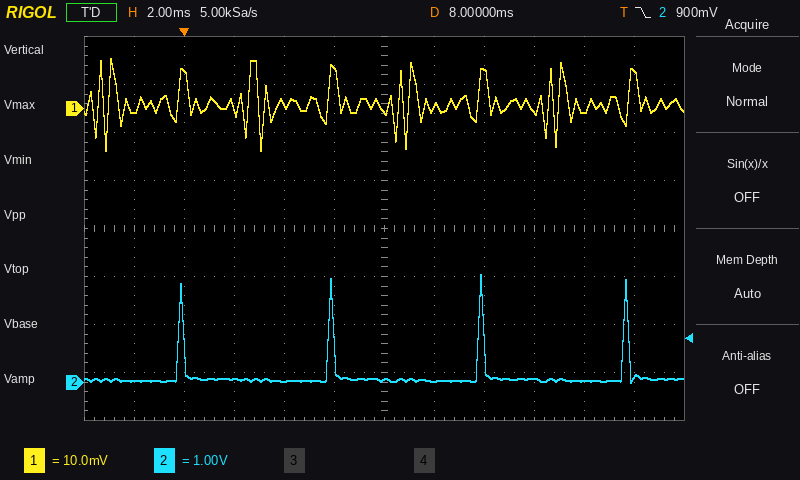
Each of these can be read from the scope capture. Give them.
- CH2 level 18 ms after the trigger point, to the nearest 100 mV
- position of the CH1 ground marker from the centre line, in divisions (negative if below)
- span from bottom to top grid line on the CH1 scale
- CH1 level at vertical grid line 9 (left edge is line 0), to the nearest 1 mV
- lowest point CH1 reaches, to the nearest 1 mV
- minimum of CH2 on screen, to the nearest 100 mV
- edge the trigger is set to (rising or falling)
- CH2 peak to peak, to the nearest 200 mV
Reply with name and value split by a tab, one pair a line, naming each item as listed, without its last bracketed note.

CH2 level 18 ms after the trigger point, to the nearest 100 mV	100 mV
position of the CH1 ground marker from the centre line, in divisions	+2.5 div
span from bottom to top grid line on the CH1 scale	80 mV
CH1 level at vertical grid line 9 (left edge is line 0), to the nearest 1 mV	-1 mV
lowest point CH1 reaches, to the nearest 1 mV	-9 mV
minimum of CH2 on screen, to the nearest 100 mV	0.0 V
edge the trigger is set to	falling
CH2 peak to peak, to the nearest 200 mV	2.2 V
